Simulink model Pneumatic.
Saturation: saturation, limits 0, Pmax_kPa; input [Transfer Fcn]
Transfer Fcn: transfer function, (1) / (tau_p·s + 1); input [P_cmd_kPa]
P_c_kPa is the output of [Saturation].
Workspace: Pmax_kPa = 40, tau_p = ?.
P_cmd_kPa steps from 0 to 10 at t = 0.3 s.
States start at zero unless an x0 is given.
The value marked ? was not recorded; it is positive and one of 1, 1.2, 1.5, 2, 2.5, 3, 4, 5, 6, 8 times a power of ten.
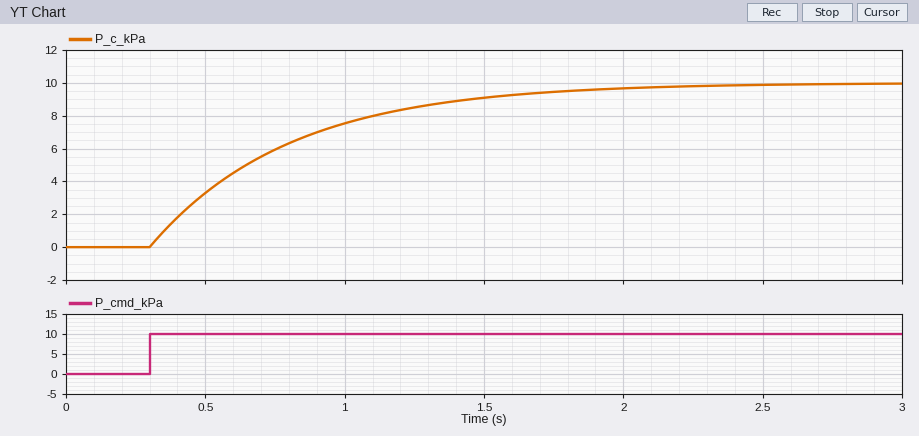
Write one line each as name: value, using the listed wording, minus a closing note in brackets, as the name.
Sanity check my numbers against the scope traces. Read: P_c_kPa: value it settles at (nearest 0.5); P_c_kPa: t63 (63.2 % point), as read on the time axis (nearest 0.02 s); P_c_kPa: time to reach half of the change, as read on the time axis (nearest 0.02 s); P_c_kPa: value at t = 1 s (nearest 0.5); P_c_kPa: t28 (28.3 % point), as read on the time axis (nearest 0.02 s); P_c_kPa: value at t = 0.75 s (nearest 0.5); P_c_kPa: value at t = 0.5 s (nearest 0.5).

P_c_kPa: value it settles at: 10.0
P_c_kPa: t63 (63.2 % point), as read on the time axis: 0.80 s
P_c_kPa: time to reach half of the change, as read on the time axis: 0.64 s
P_c_kPa: value at t = 1 s: 7.5
P_c_kPa: t28 (28.3 % point), as read on the time axis: 0.46 s
P_c_kPa: value at t = 0.75 s: 6.0
P_c_kPa: value at t = 0.5 s: 3.5
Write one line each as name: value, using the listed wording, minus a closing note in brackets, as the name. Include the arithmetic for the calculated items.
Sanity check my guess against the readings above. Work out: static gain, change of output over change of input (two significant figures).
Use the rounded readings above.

static gain, change of output over change of input: (10 - 0) / (10 - 0) = 1.0
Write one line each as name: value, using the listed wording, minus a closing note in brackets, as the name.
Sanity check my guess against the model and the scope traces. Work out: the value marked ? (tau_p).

the value marked ?: 0.5
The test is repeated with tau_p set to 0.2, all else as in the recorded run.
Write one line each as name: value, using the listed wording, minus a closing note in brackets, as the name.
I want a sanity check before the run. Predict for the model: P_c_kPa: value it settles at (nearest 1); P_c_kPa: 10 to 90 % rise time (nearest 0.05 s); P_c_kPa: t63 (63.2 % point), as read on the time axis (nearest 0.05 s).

P_c_kPa: value it settles at: 10
P_c_kPa: 10 to 90 % rise time: 0.45 s
P_c_kPa: t63 (63.2 % point), as read on the time axis: 0.50 s
